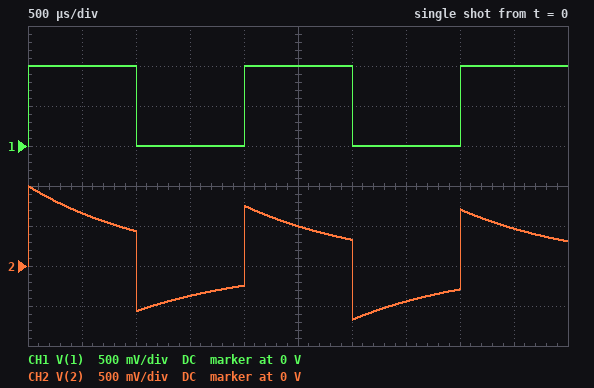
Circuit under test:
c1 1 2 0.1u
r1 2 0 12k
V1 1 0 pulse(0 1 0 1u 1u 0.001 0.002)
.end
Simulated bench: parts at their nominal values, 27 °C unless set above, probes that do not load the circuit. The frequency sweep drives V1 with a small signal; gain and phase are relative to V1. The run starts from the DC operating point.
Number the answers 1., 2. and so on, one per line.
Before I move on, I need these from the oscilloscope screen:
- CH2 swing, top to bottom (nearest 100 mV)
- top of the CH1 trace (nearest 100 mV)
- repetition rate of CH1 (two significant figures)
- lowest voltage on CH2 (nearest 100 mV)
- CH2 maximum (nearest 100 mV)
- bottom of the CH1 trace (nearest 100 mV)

1. 1.7 V
2. 1.0 V
3. 500 Hz
4. -700 mV
5. 1.0 V
6. 0 V
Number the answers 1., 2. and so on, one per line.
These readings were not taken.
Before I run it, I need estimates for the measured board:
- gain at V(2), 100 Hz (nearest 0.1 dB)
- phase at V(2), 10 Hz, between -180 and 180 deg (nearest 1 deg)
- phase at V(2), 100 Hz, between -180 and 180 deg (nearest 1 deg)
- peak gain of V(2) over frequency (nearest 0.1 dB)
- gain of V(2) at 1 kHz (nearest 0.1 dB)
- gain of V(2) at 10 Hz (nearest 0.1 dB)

1. -4.4 dB
2. 86 deg
3. 53 deg
4. 0 dB
5. -0.1 dB
6. -22.5 dB
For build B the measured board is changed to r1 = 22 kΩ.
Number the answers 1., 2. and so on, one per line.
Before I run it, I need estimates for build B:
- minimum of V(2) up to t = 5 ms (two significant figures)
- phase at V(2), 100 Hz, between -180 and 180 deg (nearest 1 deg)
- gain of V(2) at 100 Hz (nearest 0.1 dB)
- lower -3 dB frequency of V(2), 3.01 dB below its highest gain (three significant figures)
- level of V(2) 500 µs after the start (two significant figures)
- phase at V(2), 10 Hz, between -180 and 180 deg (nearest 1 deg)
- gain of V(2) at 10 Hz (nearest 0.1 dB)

1. -510 mV
2. 36 deg
3. -1.8 dB
4. 72.3 Hz
5. 800 mV
6. 82 deg
7. -17.3 dB
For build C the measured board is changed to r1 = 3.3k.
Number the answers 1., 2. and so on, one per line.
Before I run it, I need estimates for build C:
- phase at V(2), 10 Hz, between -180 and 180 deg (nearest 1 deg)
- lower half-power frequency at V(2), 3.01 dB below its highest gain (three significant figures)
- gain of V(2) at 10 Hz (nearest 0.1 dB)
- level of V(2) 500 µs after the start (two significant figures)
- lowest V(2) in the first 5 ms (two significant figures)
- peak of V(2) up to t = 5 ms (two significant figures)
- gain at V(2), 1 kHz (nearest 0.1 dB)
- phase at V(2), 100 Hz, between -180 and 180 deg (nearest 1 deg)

1. 89 deg
2. 482 Hz
3. -33.7 dB
4. 220 mV
5. -950 mV
6. 1.0 V
7. -0.9 dB
8. 78 deg
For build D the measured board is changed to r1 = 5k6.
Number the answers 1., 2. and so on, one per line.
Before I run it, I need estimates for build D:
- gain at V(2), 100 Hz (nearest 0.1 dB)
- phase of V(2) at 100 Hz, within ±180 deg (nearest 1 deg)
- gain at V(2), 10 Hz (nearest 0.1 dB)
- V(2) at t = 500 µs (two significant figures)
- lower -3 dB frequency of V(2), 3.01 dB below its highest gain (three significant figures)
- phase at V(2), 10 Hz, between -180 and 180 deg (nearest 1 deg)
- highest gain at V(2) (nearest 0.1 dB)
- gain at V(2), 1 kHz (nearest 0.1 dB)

1. -9.6 dB
2. 71 deg
3. -29.1 dB
4. 410 mV
5. 284 Hz
6. 88 deg
7. 0 dB
8. -0.3 dB
